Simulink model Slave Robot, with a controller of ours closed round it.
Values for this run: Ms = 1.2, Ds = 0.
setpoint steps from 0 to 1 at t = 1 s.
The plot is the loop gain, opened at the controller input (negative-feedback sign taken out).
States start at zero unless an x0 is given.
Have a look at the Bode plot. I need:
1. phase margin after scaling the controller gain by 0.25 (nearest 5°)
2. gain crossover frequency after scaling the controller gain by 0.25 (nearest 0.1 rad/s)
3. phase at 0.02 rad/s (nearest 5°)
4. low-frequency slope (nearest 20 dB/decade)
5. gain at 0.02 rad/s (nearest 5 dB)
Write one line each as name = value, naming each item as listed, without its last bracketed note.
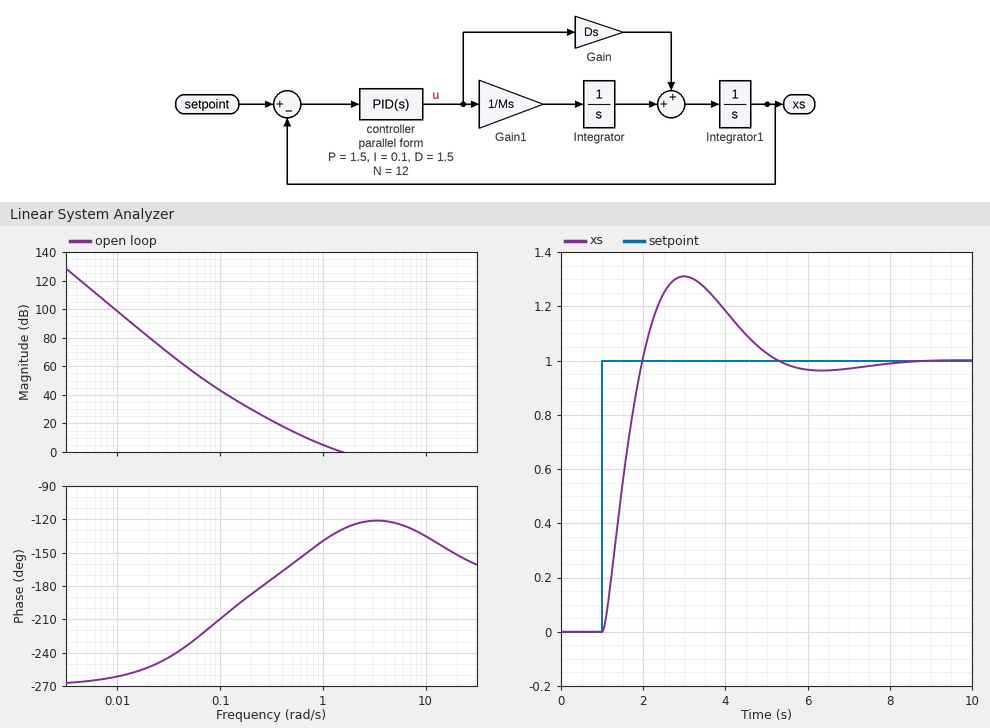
phase margin after scaling the controller gain by 0.25 = 25°
gain crossover frequency after scaling the controller gain by 0.25 = 0.6 rad/s
phase at 0.02 rad/s = -255°
low-frequency slope = -60 dB/decade
gain at 0.02 rad/s = 80 dB
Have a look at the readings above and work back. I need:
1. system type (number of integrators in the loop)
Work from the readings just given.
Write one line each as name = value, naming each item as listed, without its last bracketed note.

system type = 3
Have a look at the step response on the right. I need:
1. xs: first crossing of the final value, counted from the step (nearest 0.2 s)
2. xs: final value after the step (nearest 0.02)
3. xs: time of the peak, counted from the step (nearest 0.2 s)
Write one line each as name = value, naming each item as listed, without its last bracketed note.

xs: first crossing of the final value, counted from the step = 1.0 s
xs: final value after the step = 1.00
xs: time of the peak, counted from the step = 2.0 s
